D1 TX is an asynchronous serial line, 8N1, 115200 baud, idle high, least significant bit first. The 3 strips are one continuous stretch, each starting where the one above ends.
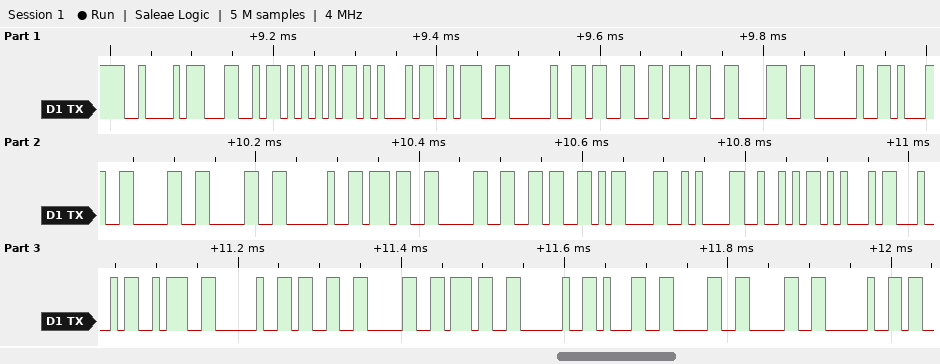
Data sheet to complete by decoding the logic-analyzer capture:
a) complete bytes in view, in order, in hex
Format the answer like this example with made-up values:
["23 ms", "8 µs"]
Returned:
["42 4C 55 45 3A 20 33 37 38 20 31 30 30 20 37 30 36 0D 0A 52 45 44 3A 20 33 30 37 20 31 30 30 20"]
